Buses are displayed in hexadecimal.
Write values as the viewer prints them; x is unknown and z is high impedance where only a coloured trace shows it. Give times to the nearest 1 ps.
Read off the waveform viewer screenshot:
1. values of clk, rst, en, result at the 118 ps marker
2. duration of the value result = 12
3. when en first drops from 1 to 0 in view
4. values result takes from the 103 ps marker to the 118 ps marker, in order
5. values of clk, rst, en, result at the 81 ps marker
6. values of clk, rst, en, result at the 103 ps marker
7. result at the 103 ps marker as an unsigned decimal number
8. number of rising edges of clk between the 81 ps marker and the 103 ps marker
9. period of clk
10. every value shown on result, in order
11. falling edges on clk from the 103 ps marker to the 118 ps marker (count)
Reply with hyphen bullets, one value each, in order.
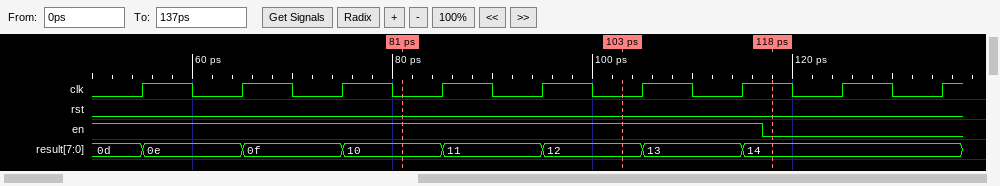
- clk=1, rst=0, en=0, result=14
- 10 ps
- 117 ps
- 12, 13, 14
- clk=0, rst=0, en=1, result=10
- clk=0, rst=0, en=1, result=12
- 18
- 2
- 10 ps
- 0d, 0e, 0f, 10, 11, 12, 13, 14
- 1
